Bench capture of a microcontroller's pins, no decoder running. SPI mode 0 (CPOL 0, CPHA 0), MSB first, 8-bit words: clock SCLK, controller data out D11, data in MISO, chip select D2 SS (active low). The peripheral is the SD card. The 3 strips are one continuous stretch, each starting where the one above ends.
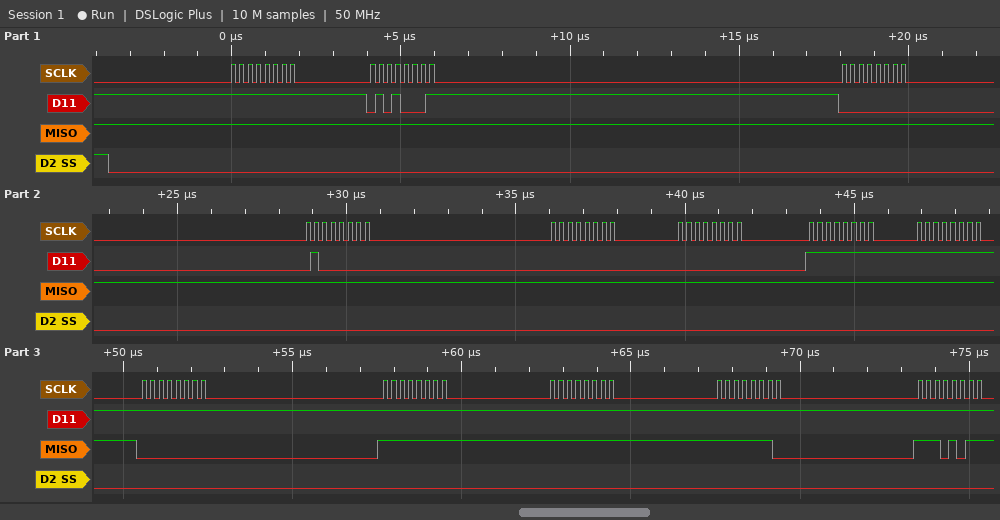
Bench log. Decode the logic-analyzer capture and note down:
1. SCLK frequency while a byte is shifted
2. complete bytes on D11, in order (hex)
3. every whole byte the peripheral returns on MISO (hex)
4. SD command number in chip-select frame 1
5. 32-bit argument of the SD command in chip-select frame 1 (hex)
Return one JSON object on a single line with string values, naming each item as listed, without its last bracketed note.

{"SCLK frequency while a byte is shifted": "4 MHz", "complete bytes on D11, in order": "0xFF 0x51 0x00 0x40 0x00 0x00 0xFF 0xFF 0xFF 0xFF 0xFF 0xFF 0xFF", "every whole byte the peripheral returns on MISO": "0xFF 0xFF 0xFF 0xFF 0xFF 0xFF 0xFF 0xFF 0x00 0xFF 0xFF 0xFE 0xEB", "SD command number in chip-select frame 1": "CMD17", "32-bit argument of the SD command in chip-select frame 1": "0x00400000"}
